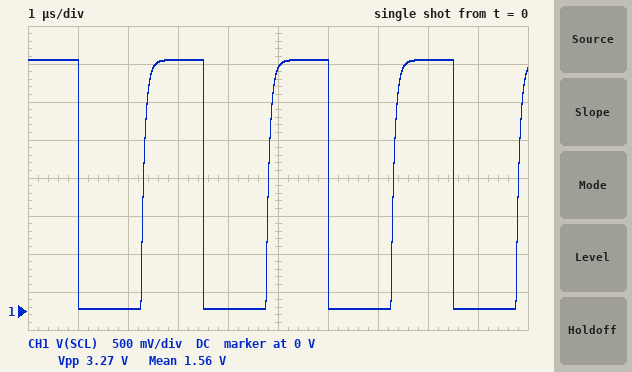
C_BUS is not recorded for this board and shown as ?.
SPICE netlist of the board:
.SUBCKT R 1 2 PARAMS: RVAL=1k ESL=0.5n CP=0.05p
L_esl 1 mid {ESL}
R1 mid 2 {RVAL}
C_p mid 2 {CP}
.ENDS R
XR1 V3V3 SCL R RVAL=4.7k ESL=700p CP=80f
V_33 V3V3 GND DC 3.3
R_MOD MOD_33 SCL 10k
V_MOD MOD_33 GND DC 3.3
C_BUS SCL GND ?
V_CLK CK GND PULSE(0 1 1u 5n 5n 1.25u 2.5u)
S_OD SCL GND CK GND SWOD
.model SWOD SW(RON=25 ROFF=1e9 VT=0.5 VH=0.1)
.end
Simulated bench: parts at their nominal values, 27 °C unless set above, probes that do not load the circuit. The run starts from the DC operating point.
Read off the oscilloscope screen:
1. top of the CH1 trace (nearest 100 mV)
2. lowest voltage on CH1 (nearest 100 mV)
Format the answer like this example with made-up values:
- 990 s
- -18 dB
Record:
- 3.3 V
- 0 V
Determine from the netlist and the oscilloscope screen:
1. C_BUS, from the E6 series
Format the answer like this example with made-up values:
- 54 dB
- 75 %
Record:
- 22 pF
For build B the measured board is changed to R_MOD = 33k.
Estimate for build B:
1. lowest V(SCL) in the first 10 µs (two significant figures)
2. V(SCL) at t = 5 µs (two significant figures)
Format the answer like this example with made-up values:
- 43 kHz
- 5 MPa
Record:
- 20 mV
- 3.1 V
